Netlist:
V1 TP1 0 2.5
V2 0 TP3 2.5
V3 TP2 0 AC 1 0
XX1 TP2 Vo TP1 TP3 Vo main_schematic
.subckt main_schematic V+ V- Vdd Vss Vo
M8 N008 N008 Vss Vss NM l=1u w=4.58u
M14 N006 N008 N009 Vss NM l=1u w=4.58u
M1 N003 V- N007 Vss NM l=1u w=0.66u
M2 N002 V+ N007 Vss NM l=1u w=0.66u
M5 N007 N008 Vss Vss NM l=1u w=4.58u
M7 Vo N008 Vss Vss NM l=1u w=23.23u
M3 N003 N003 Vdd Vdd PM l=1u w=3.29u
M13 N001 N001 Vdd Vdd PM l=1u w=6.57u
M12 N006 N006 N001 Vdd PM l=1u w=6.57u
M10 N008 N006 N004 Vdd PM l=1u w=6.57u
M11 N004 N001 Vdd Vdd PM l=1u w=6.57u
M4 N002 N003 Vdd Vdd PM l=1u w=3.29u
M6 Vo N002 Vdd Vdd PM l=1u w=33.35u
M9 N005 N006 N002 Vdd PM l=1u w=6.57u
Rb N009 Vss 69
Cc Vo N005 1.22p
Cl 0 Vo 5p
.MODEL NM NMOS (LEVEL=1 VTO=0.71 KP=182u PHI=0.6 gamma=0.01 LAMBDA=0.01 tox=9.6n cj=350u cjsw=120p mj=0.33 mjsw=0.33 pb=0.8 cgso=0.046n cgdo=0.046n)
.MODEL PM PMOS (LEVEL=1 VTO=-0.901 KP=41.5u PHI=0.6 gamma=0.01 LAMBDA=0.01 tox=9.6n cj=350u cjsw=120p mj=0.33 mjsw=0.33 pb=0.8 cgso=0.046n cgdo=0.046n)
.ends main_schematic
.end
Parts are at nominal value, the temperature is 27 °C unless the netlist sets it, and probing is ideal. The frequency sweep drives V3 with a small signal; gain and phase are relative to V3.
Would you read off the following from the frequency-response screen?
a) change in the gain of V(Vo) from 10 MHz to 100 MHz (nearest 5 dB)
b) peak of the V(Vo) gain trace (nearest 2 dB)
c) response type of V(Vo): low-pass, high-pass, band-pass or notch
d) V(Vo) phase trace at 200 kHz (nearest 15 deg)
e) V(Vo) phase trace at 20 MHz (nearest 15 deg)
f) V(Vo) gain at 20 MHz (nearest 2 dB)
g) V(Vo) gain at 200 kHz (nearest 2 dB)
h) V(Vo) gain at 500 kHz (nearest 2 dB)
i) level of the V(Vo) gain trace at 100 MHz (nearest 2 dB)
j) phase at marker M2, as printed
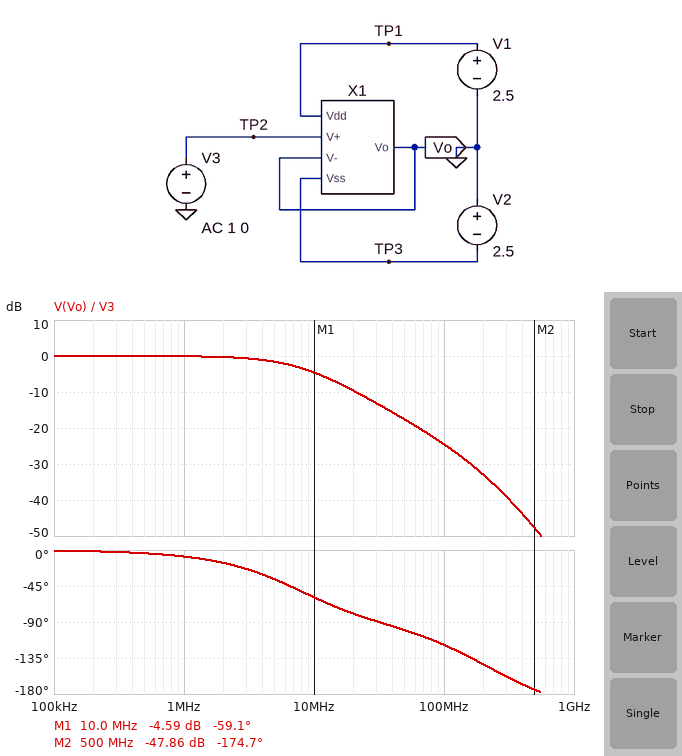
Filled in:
-20 dB
0 dB
low-pass
0 deg
-75 deg
-10 dB
0 dB
0 dB
-24 dB
-174.7 deg
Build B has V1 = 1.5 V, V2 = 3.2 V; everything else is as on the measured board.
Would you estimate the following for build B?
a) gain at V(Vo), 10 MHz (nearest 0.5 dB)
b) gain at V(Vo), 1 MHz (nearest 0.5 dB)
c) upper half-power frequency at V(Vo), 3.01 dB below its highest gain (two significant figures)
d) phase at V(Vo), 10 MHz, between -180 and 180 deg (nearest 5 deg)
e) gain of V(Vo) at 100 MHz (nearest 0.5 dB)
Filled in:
-5.5 dB
0 dB
6.5 MHz
-65 deg
-26.0 dB
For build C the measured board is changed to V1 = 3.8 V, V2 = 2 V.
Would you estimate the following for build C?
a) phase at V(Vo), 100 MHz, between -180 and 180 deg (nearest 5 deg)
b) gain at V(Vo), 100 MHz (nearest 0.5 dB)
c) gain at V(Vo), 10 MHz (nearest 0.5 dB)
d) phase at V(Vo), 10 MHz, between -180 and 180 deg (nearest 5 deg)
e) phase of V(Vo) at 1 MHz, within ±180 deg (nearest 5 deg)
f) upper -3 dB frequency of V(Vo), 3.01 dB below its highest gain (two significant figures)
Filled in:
-110 deg
-21.5 dB
-3.0 dB
-50 deg
-5 deg
9.8 MHz
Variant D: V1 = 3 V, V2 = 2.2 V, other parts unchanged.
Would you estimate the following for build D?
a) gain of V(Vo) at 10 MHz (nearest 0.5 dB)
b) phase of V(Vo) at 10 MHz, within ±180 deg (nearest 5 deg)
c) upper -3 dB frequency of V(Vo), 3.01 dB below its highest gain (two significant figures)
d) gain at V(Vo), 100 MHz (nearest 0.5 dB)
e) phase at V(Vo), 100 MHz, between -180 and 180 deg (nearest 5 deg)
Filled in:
-4.0 dB
-55 deg
8.0 MHz
-23.5 dB
-115 deg
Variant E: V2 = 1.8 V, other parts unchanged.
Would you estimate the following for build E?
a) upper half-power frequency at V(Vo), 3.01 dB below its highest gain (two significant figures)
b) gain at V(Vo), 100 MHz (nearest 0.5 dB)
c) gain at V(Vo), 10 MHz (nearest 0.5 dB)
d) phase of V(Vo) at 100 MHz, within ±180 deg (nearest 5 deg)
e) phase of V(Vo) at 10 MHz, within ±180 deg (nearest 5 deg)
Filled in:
5.3 MHz
-28.5 dB
-7.0 dB
-130 deg
-70 deg
